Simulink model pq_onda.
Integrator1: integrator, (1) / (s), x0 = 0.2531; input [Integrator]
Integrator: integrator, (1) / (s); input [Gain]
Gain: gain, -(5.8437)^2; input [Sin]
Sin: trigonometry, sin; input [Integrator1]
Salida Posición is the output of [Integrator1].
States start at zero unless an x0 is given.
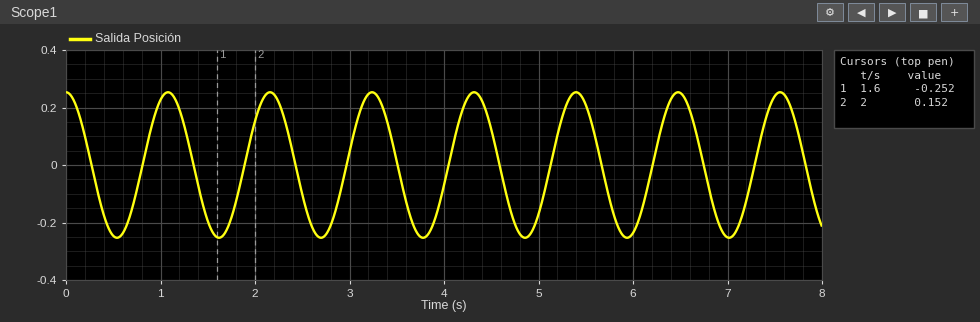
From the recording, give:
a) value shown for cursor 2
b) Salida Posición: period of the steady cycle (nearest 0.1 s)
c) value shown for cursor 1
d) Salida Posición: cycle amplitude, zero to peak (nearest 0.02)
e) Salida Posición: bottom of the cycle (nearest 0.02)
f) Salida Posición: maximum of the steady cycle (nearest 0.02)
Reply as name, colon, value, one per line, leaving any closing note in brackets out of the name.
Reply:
value shown for cursor 2: 0.152
Salida Posición: period of the steady cycle: 1.1 s
value shown for cursor 1: -0.252
Salida Posición: cycle amplitude, zero to peak: 0.26
Salida Posición: bottom of the cycle: -0.26
Salida Posición: maximum of the steady cycle: 0.26
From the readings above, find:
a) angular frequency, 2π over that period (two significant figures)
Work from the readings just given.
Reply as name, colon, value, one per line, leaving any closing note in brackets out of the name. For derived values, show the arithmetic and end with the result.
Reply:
angular frequency, 2π over that period: 2π / 1.1 = 5.7 rad/s
